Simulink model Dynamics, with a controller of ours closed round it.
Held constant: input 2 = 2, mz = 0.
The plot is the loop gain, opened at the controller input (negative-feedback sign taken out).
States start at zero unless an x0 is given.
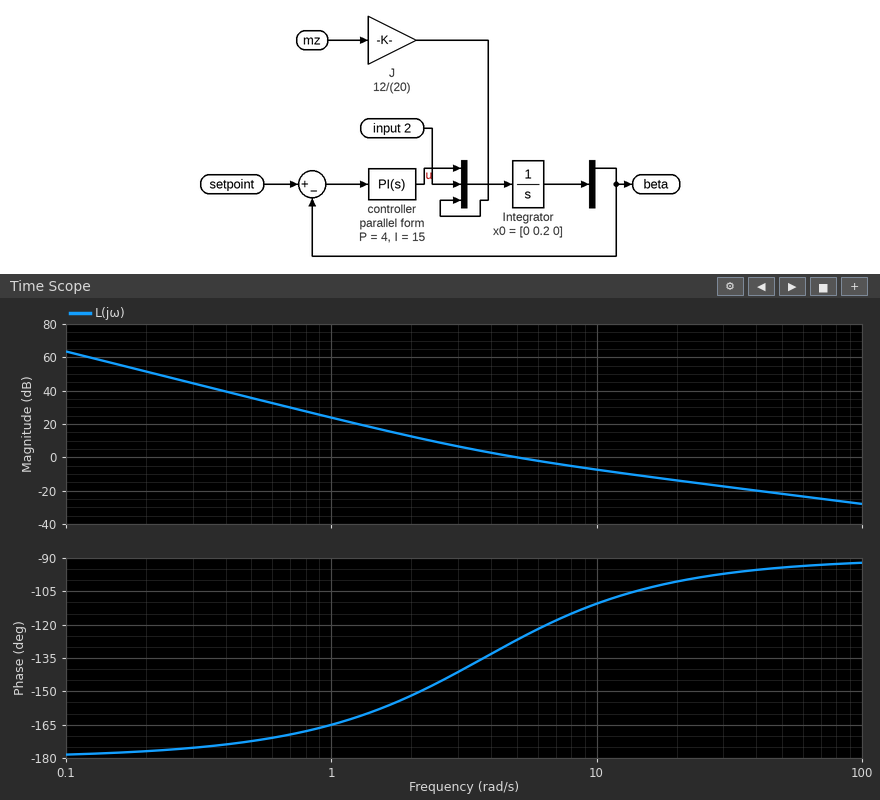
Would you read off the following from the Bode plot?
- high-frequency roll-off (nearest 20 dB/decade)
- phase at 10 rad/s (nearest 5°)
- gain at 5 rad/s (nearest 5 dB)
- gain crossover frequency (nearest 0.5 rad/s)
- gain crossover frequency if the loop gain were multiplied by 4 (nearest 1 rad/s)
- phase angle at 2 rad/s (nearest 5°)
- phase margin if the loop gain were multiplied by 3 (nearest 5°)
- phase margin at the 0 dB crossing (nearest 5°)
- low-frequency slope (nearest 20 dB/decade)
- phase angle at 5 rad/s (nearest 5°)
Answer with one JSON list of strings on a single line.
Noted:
["-20 dB/decade", "-110°", "0 dB", "5.0 rad/s", "16 rad/s", "-150°", "75°", "55°", "-40 dB/decade", "-125°"]
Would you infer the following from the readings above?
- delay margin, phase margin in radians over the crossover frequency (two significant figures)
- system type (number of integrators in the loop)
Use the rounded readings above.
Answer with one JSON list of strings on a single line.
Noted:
["0.19 s", "2"]
